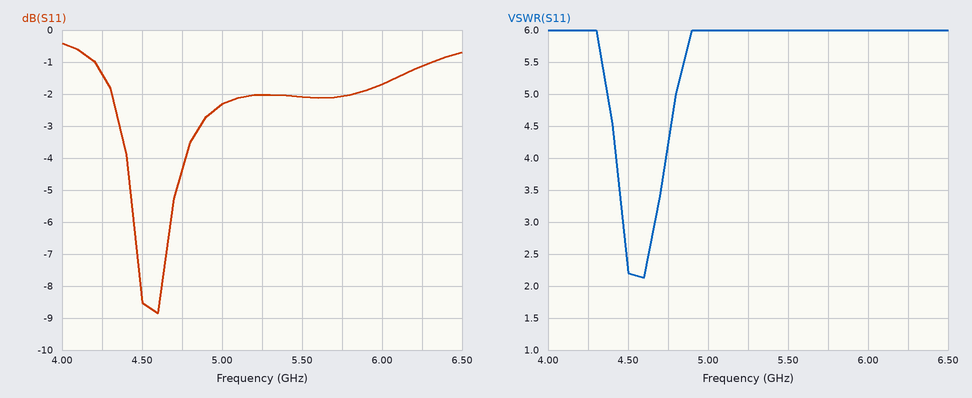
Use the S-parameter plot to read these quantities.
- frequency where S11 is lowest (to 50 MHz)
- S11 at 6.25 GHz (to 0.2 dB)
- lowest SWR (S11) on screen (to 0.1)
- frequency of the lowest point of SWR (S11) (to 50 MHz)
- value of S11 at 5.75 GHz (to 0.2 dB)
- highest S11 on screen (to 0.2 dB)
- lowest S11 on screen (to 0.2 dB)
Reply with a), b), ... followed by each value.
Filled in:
a) 4.60 GHz
b) -1.2 dB
c) 2.1
d) 4.60 GHz
e) -2.0 dB
f) -0.4 dB
g) -8.8 dB
